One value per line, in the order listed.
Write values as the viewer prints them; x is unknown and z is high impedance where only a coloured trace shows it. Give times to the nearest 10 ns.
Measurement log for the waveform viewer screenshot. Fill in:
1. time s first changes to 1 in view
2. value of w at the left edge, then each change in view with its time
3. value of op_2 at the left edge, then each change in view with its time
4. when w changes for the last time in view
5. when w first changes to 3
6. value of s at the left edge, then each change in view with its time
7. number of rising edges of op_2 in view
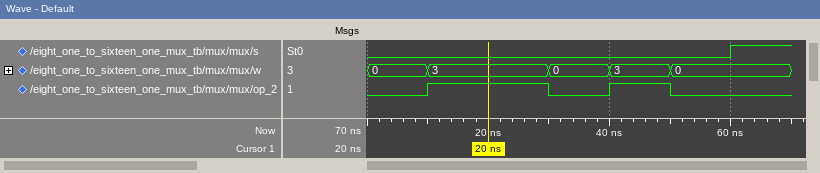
60 ns
0, 3 at 10 ns, 0 at 30 ns, 3 at 40 ns, 0 at 50 ns
0, 1 at 10 ns, 0 at 30 ns, 1 at 40 ns, 0 at 50 ns
50 ns
10 ns
0, 1 at 60 ns
2
